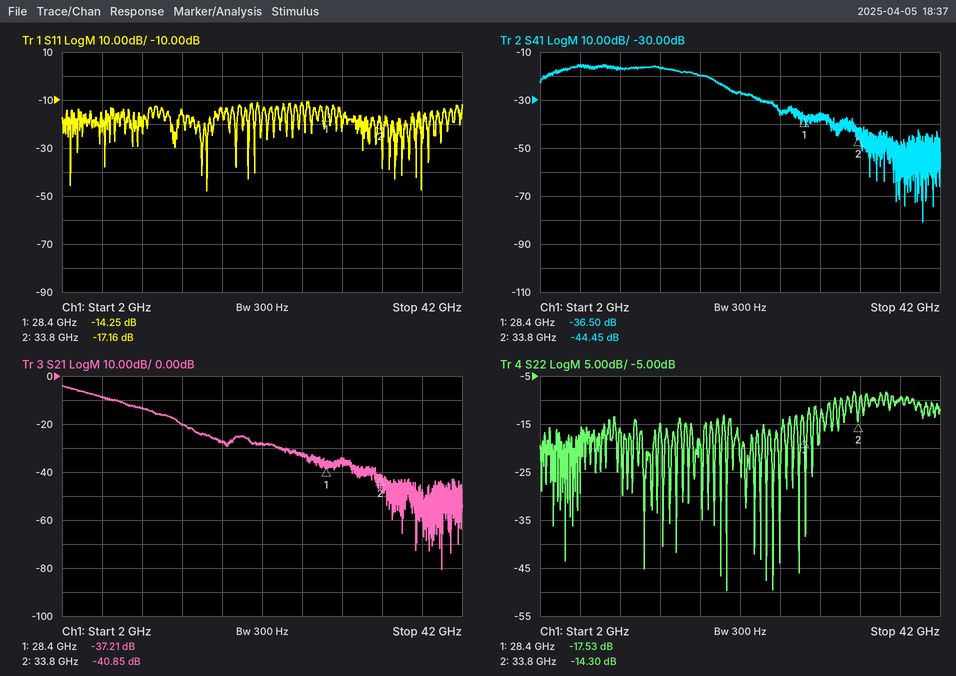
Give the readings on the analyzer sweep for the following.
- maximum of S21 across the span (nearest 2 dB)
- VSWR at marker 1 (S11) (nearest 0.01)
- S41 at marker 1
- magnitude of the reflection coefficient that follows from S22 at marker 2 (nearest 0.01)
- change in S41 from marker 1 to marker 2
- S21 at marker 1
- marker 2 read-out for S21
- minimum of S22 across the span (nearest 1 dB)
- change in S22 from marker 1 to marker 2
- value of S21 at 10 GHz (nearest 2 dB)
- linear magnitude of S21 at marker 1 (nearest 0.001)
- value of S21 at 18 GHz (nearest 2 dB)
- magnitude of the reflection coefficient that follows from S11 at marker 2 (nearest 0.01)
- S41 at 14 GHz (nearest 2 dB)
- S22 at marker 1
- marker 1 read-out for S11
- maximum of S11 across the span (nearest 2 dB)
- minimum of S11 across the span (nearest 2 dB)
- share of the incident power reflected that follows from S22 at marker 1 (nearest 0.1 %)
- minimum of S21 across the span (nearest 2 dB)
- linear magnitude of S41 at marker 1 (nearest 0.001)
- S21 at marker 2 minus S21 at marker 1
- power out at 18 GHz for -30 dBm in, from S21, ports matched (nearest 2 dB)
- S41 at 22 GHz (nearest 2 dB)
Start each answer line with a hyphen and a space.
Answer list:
- -4 dB
- 1.48
- -36.50 dB
- 0.19
- -7.95 dB
- -37.21 dB
- -40.85 dB
- -50 dB
- 3.23 dB
- -14 dB
- 0.014
- -28 dB
- 0.14
- -16 dB
- -17.53 dB
- -14.25 dB
- -10 dB
- -48 dB
- 1.8 %
- -80 dB
- 0.015
- -3.64 dB
- -58 dBm
- -26 dB
